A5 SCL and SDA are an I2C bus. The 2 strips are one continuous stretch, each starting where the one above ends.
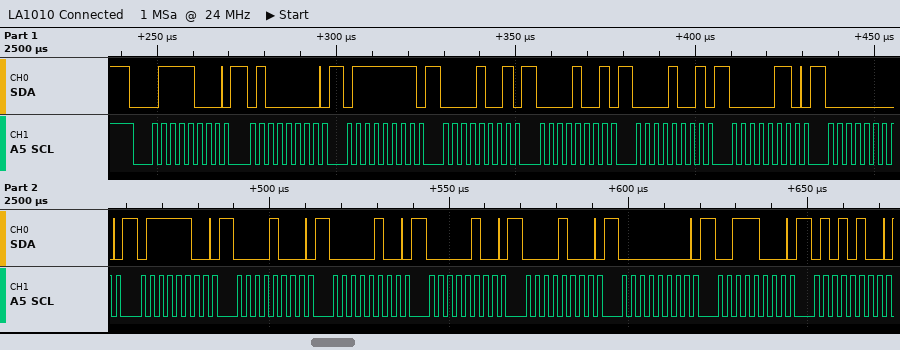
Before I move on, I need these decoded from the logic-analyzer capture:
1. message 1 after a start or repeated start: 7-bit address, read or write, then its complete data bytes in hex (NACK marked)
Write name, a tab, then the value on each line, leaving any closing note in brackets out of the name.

message 1 after a start or repeated start: 7-bit address, read or write, then its complete data bytes in hex	0x3C write: 40 7F 09 09 09 06 00 7C 08 04 04 08 00 38 54
